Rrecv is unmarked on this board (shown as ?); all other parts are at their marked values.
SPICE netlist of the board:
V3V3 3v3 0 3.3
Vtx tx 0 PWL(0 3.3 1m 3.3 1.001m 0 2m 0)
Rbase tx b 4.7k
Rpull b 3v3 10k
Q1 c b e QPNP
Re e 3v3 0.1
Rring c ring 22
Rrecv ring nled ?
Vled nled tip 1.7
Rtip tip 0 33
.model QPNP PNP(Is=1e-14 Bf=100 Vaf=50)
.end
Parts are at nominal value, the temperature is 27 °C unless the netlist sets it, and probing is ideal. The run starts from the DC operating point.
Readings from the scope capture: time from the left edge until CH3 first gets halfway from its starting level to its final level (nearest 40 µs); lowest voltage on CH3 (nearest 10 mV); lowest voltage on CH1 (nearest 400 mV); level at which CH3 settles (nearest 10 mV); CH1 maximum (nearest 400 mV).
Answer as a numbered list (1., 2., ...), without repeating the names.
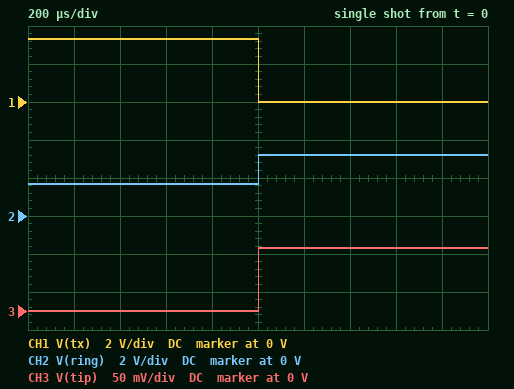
1. 1.00 ms
2. 0 V
3. 0 V
4. 80 mV
5. 3.2 V
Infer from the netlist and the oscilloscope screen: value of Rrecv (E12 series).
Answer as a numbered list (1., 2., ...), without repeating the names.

1. 560 Ω
